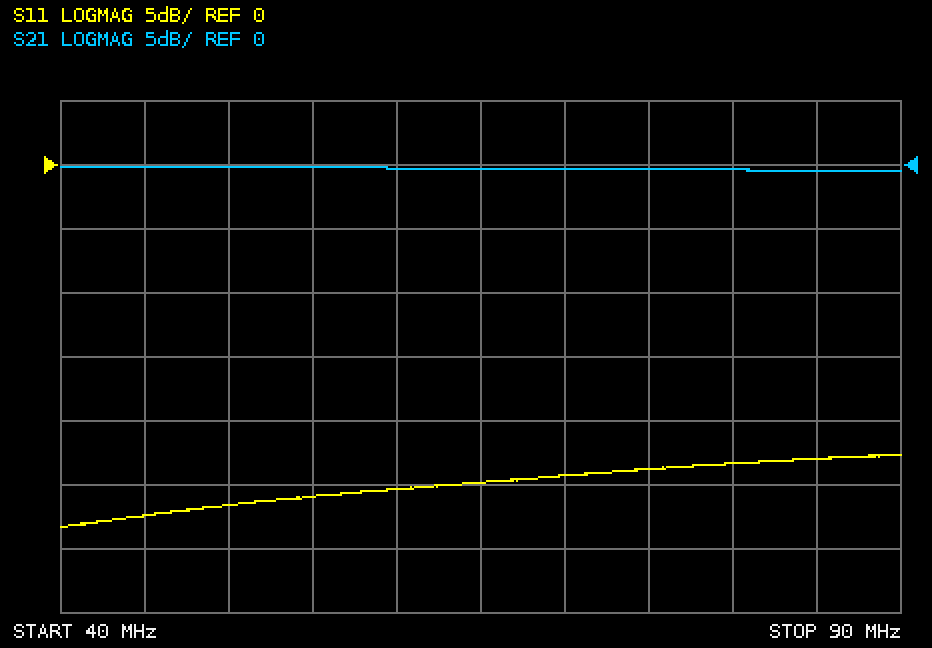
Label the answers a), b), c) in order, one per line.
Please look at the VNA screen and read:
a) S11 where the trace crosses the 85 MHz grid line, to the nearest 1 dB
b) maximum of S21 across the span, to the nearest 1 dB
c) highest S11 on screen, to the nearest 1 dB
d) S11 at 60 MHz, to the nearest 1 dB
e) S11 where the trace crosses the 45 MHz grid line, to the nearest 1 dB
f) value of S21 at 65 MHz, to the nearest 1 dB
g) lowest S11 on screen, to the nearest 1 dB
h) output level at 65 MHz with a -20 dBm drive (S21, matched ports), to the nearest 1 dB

a) -23 dB
b) 0 dB
c) -23 dB
d) -25 dB
e) -27 dB
f) 0 dB
g) -28 dB
h) -20 dBm
